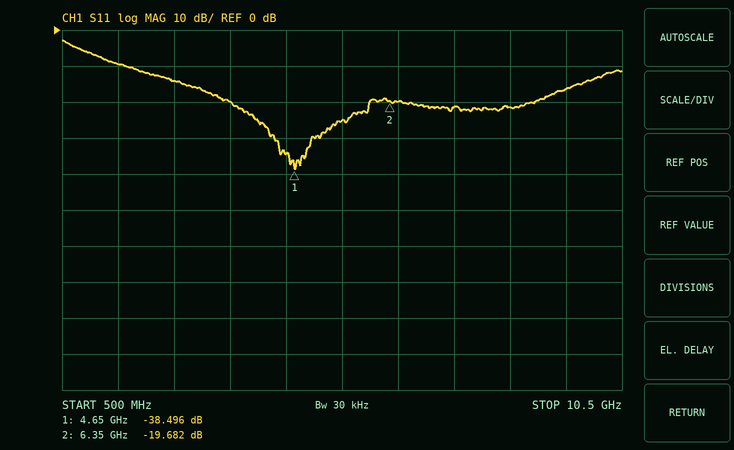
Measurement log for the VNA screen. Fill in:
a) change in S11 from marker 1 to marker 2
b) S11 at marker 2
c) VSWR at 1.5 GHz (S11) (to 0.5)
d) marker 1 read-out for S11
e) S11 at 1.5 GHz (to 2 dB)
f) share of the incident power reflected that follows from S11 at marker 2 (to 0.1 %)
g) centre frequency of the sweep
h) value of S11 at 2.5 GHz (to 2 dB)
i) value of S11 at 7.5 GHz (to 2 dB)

18.814 dB
-19.682 dB
2.0
-38.496 dB
-10 dB
1.1 %
5.5 GHz
-14 dB
-22 dB
